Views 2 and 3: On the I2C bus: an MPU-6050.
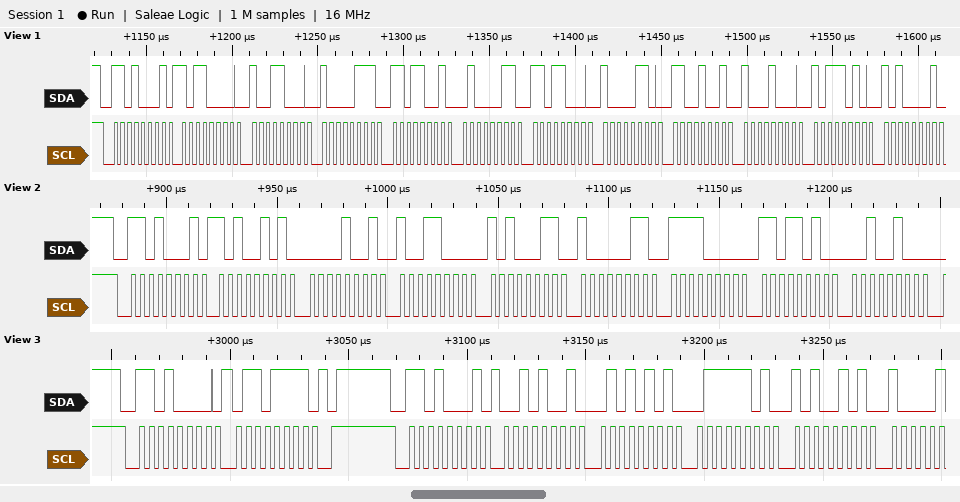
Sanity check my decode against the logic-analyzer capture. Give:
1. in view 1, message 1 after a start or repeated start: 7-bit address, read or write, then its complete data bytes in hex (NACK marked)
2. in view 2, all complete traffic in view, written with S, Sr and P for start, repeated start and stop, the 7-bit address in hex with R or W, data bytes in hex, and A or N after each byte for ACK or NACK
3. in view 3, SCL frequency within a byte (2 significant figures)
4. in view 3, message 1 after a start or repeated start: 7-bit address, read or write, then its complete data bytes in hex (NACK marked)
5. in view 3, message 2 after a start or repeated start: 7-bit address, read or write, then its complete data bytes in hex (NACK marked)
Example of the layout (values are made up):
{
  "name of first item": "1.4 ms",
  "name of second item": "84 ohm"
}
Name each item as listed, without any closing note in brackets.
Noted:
{
  "in view 1, message 1 after a start or repeated start: 7-bit address, read or write, then its complete data bytes in hex": "0x68 read: B0 98 87 D9 43 D8 86 C9 88 BA A1",
  "in view 2, all complete traffic in view, written with S, Sr and P for start, repeated start and stop, the 7-bit address in hex with R or W, data bytes in hex, and A or N after each byte for ACK or NACK": "S 68R A A5 A 09 A 98 A A3 A 83 A F0 A DA A 24 A",
  "in view 3, SCL frequency within a byte": "250 kHz",
  "in view 3, message 1 after a start or repeated start: 7-bit address, read or write, then its complete data bytes in hex": "0x68 write: 6F",
  "in view 3, message 2 after a start or repeated start: 7-bit address, read or write, then its complete data bytes in hex": "0x68 read: 29 55 7D A5"
}
